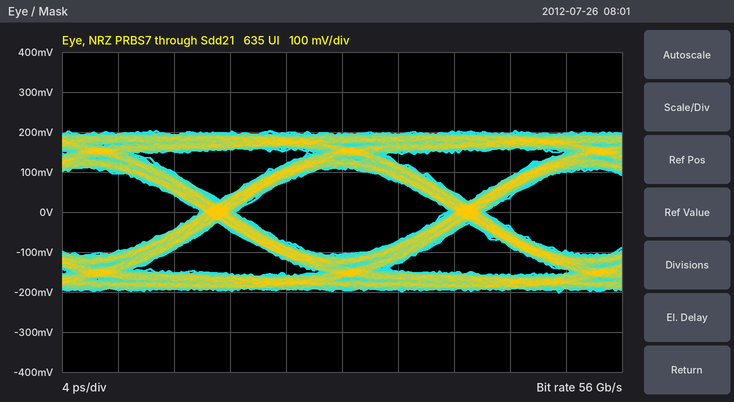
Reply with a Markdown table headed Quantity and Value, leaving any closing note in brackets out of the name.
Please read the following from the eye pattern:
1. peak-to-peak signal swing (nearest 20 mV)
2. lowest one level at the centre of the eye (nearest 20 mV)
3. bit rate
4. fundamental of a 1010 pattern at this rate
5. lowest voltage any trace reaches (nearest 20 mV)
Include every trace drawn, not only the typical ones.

| Quantity | Value |
|---|---|
| peak-to-peak signal swing | 400 mV |
| lowest one level at the centre of the eye | 100 mV |
| bit rate | 56 Gb/s |
| fundamental of a 1010 pattern at this rate | 28 GHz |
| lowest voltage any trace reaches | -200 mV |
